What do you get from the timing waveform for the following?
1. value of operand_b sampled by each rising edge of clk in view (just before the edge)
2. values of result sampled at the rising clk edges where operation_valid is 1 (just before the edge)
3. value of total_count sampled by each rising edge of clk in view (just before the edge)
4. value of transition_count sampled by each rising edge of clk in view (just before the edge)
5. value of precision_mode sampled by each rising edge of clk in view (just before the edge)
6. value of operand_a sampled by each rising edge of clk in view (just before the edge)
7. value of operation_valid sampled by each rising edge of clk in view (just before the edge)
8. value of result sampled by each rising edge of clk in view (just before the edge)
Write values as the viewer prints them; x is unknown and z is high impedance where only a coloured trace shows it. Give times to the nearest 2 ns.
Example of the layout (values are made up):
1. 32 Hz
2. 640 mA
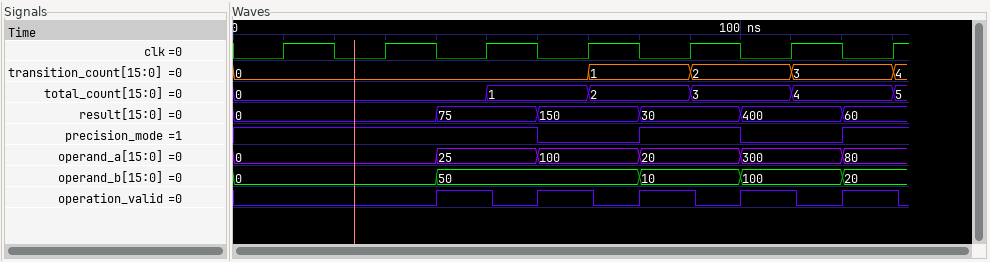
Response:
1. 0, 0, 50, 50, 10, 100, 20
2. 75, 150, 30, 400, 60
3. 0, 0, 0, 1, 2, 3, 4
4. 0, 0, 0, 0, 1, 2, 3
5. 1 1 1 0 1 0 1
6. 0, 0, 25, 100, 20, 300, 80
7. 0 0 1 1 1 1 1
8. 0, 0, 75, 150, 30, 400, 60
